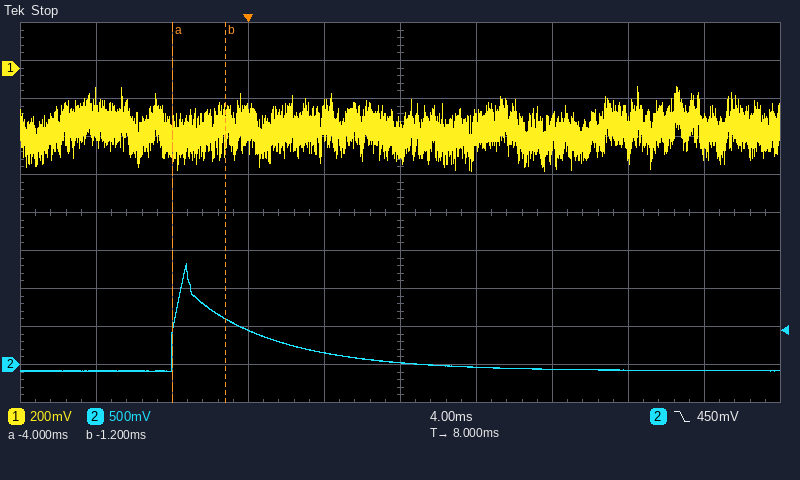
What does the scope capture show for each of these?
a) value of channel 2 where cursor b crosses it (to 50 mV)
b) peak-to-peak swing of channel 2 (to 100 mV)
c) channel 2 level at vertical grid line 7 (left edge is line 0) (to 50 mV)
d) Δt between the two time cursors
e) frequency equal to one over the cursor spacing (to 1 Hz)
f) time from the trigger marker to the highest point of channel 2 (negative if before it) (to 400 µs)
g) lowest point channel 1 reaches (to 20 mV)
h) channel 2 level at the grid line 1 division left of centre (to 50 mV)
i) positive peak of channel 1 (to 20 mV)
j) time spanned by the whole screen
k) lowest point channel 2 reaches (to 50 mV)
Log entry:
600 mV
1.40 V
-50 mV
2.8 ms
357 Hz
-3.2 ms
-540 mV
150 mV
-100 mV
40 ms
-100 mV
